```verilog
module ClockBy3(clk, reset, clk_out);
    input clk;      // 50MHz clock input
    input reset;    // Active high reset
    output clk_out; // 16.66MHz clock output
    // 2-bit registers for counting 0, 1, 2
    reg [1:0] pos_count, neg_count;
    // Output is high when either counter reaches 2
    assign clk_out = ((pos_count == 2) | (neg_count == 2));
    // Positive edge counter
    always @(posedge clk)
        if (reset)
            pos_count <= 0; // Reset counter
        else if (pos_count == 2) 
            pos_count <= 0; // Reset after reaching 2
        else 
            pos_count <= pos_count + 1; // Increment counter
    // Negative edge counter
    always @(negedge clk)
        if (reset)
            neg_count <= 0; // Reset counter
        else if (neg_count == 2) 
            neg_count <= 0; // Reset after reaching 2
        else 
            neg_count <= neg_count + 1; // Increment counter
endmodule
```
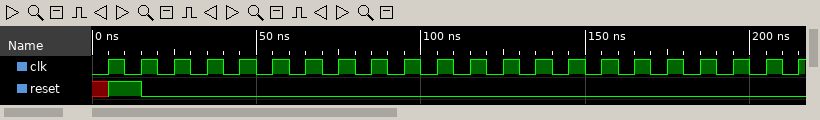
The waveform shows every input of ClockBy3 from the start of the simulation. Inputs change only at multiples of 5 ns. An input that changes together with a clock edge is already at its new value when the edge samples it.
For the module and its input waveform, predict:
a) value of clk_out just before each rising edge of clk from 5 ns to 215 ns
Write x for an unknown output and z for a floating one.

x 0 0 1 0 0 1 0 0 1 0 0 1 0 0 1 0 0 1 0 0 1
